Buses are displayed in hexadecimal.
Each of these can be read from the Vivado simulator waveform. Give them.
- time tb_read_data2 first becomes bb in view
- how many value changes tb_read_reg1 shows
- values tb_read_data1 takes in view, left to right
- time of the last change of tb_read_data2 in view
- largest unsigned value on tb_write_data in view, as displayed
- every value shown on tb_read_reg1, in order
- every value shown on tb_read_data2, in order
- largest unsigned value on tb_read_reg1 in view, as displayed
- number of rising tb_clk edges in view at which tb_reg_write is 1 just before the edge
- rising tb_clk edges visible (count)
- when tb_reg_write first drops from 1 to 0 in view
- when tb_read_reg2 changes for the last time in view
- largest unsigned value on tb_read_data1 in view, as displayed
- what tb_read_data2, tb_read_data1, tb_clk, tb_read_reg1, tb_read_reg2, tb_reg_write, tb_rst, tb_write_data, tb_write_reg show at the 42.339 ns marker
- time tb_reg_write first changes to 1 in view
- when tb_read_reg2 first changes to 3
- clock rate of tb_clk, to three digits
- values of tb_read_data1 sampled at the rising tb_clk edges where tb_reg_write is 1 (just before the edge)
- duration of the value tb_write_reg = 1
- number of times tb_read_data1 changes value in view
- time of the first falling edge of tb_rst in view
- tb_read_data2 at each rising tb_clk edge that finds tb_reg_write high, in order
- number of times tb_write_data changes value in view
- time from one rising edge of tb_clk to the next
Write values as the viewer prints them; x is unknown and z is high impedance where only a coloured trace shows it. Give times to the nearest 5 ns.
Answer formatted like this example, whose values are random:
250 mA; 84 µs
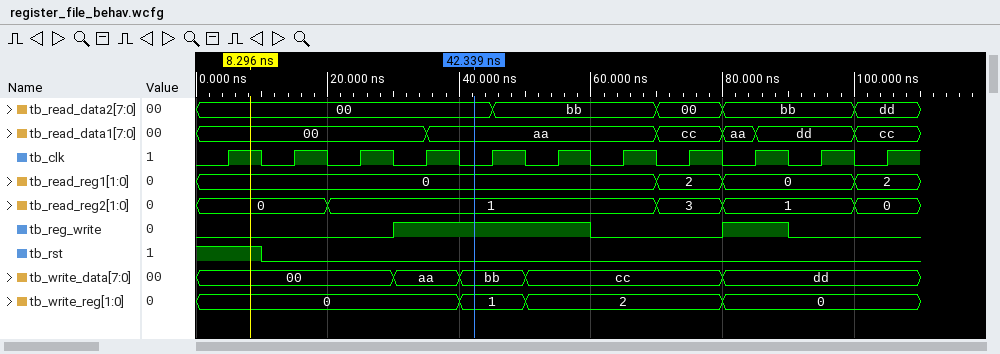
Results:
45 ns; 3; 00, aa, cc, aa, dd, cc; 100 ns; dd; 0, 2, 0, 2; 00, bb, 00, bb, dd; 2; 4; 11; 60 ns; 100 ns; dd; tb_read_data2=00, tb_read_data1=aa, tb_clk=0, tb_read_reg1=0, tb_read_reg2=1, tb_reg_write=1, tb_rst=0, tb_write_data=bb, tb_write_reg=1; 30 ns; 70 ns; 100 MHz; 00, aa, aa, aa; 10 ns; 5; 10 ns; 00, 00, bb, bb; 4; 10 ns
